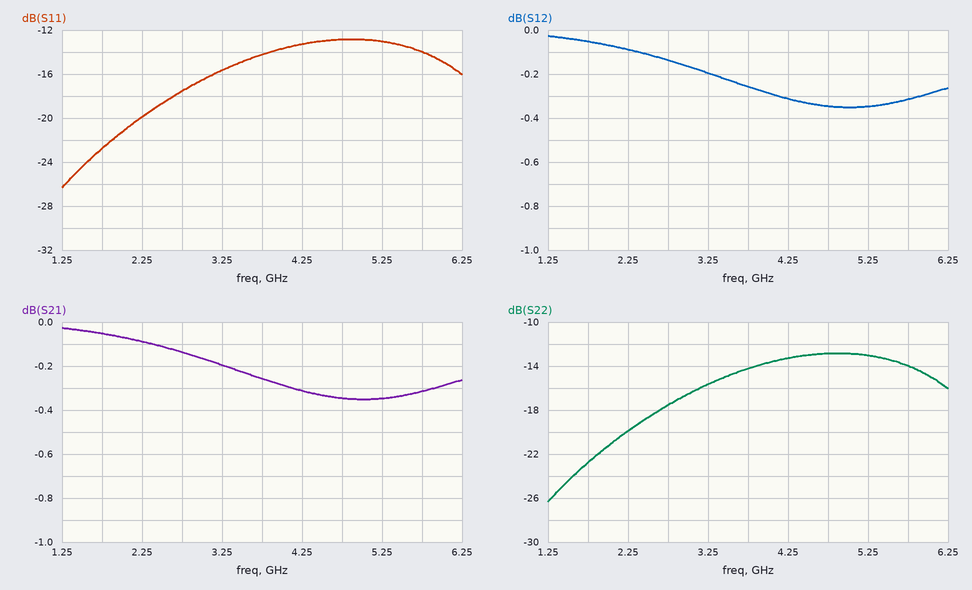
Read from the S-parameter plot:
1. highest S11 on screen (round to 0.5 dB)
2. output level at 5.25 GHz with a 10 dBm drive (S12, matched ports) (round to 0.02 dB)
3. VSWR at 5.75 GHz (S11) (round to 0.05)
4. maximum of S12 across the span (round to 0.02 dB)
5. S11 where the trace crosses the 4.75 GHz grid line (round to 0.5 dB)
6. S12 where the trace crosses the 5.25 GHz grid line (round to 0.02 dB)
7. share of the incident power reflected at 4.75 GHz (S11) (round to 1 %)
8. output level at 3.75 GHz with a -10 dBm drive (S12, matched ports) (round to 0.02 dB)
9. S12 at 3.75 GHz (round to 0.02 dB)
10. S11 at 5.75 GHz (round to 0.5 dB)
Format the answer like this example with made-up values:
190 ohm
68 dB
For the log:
-13.0 dB
9.66 dBm
1.50
-0.02 dB
-13.0 dB
-0.34 dB
5 %
-10.26 dBm
-0.26 dB
-14.0 dB
